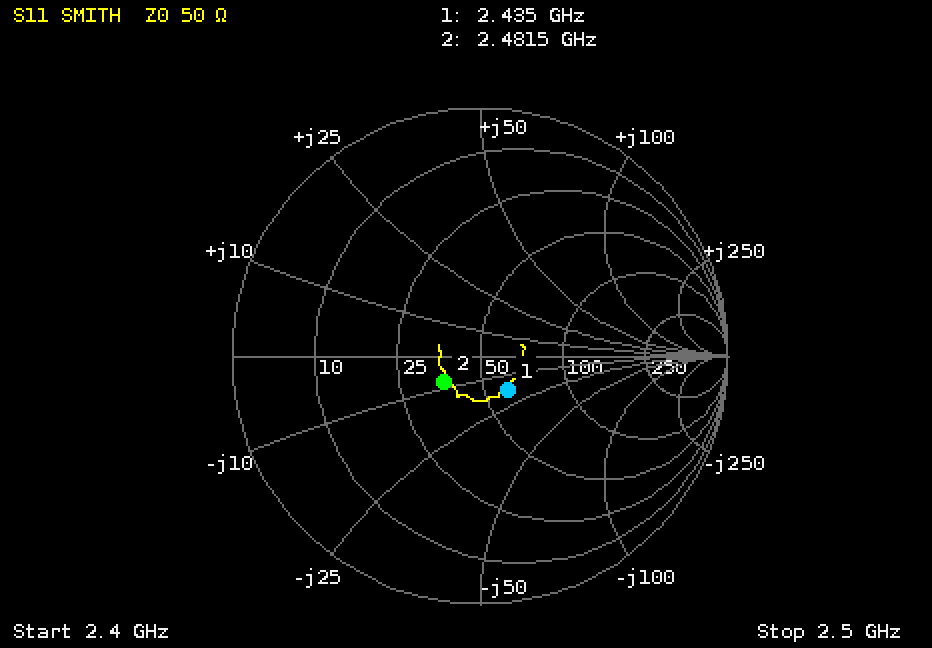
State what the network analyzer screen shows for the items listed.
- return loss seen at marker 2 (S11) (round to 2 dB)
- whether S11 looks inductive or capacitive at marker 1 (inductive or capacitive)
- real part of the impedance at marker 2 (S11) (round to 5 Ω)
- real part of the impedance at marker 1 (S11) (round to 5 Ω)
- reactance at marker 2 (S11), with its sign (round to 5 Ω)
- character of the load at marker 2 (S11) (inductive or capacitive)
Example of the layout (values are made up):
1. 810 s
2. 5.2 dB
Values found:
1. 14 dB
2. capacitive
3. 35 Ω
4. 60 Ω
5. -10 Ω
6. capacitive
